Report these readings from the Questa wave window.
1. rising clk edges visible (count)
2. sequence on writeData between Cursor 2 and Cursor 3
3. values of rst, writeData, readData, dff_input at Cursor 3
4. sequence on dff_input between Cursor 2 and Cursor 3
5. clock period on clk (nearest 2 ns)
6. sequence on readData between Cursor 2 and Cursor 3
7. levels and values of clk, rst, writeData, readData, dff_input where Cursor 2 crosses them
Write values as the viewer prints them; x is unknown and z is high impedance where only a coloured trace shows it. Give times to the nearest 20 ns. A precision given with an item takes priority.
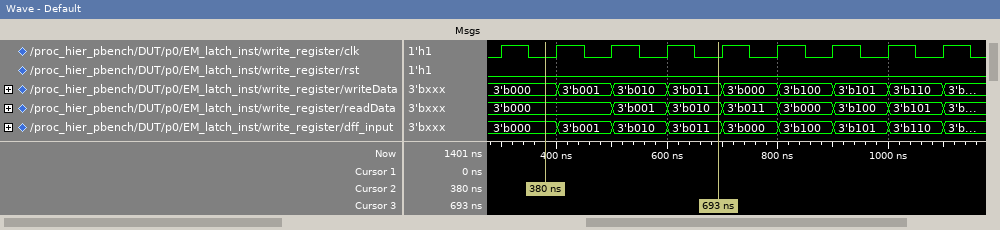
9
3'b000, 3'b001, 3'b010, 3'b011
rst=0, writeData=3'b011, readData=3'b010, dff_input=3'b011
3'b000, 3'b001, 3'b010, 3'b011
100 ns
3'b000, 3'b001, 3'b010
clk=0, rst=0, writeData=3'b000, readData=3'b000, dff_input=3'b000
